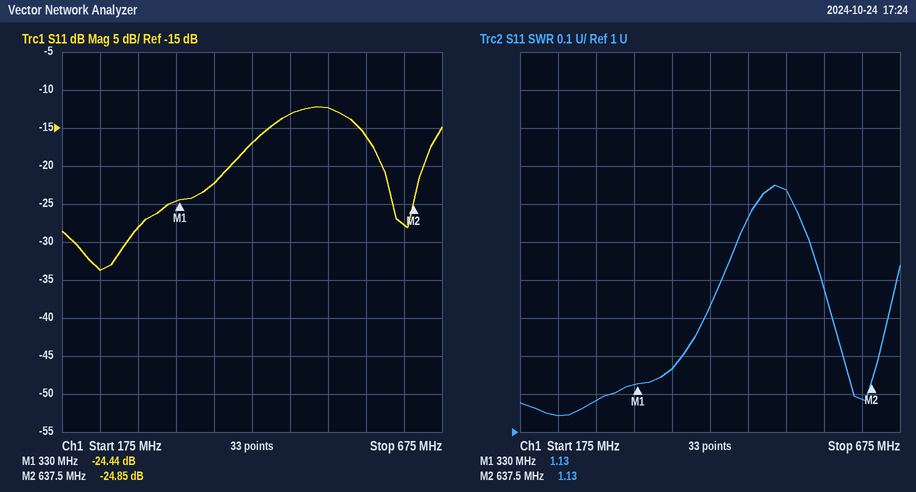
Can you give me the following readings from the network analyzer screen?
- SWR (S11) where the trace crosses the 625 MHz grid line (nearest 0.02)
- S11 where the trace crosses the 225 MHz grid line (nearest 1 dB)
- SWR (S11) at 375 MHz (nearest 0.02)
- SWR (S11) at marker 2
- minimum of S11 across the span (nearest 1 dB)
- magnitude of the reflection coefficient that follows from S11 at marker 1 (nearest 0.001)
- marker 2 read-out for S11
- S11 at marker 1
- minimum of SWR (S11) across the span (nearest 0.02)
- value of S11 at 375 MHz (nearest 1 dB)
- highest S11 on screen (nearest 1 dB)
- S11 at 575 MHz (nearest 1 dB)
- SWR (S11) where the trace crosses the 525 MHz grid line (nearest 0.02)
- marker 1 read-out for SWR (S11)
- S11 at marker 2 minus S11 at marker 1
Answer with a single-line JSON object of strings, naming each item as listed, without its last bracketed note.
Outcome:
{"SWR (S11) where the trace crosses the 625 MHz grid line": "1.08", "S11 where the trace crosses the 225 MHz grid line": "-34 dB", "SWR (S11) at 375 MHz": "1.16", "SWR (S11) at marker 2": "1.13", "minimum of S11 across the span": "-34 dB", "magnitude of the reflection coefficient that follows from S11 at marker 1": "0.060", "marker 2 read-out for S11": "-24.85 dB", "S11 at marker 1": "-24.44 dB", "minimum of SWR (S11) across the span": "1.04", "value of S11 at 375 MHz": "-22 dB", "highest S11 on screen": "-12 dB", "S11 at 575 MHz": "-16 dB", "SWR (S11) where the trace crosses the 525 MHz grid line": "1.64", "marker 1 read-out for SWR": "1.13", "S11 at marker 2 minus S11 at marker 1": "-0.41 dB"}
